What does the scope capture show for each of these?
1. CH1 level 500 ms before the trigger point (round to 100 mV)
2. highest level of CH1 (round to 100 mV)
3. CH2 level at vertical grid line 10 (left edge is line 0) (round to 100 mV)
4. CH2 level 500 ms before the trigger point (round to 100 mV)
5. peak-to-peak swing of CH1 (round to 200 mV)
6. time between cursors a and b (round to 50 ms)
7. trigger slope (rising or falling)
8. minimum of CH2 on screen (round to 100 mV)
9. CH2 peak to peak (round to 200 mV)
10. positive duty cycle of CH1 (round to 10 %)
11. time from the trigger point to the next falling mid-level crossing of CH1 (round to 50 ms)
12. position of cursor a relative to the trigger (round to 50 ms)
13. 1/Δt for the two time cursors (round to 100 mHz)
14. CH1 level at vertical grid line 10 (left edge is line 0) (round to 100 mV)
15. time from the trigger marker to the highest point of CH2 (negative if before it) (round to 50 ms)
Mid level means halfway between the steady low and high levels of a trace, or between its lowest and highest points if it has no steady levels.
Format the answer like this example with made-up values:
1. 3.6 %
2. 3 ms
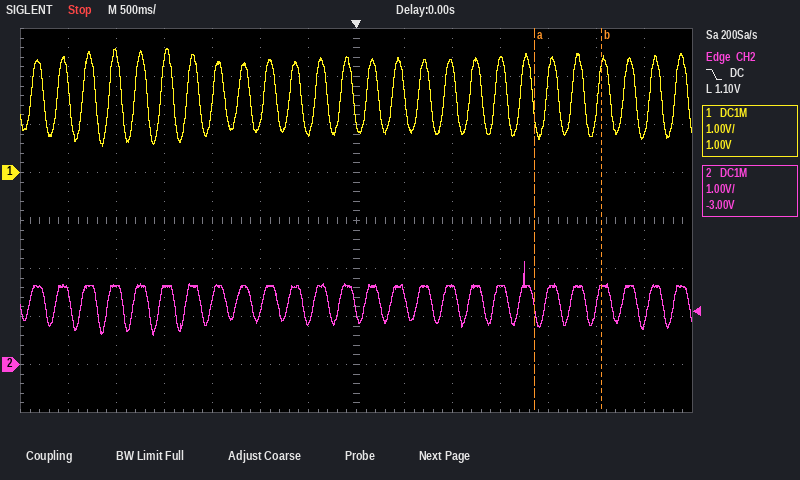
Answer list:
1. 800 mV
2. 2.6 V
3. 1.6 V
4. 900 mV
5. 2.0 V
6. 700 ms
7. falling
8. 600 mV
9. 1.6 V
10. 50 %
11. 250 ms
12. +1.85 s
13. 1.4 Hz
14. 2.3 V
15. +1.75 s
